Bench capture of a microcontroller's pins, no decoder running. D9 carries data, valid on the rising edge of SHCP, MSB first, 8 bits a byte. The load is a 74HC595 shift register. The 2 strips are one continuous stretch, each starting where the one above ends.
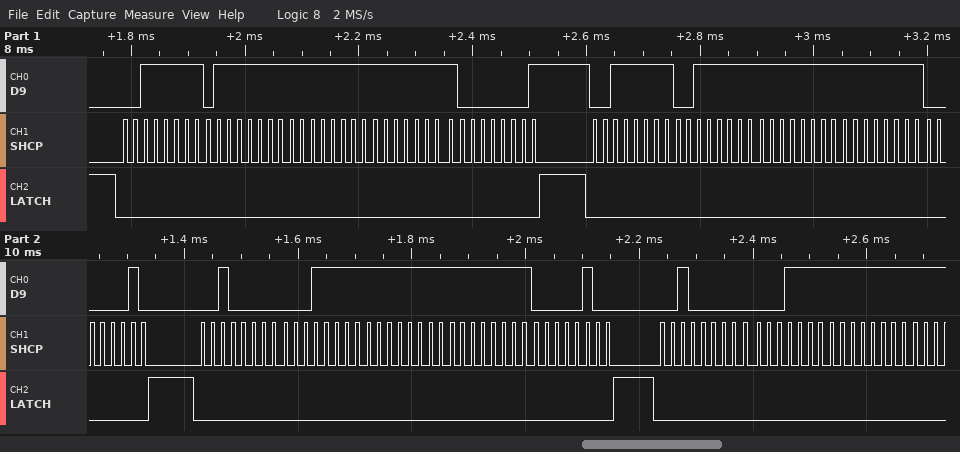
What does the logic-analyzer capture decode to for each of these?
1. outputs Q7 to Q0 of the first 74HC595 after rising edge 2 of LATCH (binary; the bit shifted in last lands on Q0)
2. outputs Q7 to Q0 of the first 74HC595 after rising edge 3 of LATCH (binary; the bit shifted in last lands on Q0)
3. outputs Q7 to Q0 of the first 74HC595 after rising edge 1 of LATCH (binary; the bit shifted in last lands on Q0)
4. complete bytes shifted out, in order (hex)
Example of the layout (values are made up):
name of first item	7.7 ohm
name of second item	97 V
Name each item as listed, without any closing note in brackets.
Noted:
outputs Q7 to Q0 of the first 74HC595 after rising edge 2 of LATCH	00000010
outputs Q7 to Q0 of the first 74HC595 after rising edge 3 of LATCH	00000100
outputs Q7 to Q0 of the first 74HC595 after rising edge 1 of LATCH	00000001
complete bytes shifted out, in order	3F 7F FF FF 01 3F 3F FF FF 02 20 1F FF FF 04 20 0F FF
